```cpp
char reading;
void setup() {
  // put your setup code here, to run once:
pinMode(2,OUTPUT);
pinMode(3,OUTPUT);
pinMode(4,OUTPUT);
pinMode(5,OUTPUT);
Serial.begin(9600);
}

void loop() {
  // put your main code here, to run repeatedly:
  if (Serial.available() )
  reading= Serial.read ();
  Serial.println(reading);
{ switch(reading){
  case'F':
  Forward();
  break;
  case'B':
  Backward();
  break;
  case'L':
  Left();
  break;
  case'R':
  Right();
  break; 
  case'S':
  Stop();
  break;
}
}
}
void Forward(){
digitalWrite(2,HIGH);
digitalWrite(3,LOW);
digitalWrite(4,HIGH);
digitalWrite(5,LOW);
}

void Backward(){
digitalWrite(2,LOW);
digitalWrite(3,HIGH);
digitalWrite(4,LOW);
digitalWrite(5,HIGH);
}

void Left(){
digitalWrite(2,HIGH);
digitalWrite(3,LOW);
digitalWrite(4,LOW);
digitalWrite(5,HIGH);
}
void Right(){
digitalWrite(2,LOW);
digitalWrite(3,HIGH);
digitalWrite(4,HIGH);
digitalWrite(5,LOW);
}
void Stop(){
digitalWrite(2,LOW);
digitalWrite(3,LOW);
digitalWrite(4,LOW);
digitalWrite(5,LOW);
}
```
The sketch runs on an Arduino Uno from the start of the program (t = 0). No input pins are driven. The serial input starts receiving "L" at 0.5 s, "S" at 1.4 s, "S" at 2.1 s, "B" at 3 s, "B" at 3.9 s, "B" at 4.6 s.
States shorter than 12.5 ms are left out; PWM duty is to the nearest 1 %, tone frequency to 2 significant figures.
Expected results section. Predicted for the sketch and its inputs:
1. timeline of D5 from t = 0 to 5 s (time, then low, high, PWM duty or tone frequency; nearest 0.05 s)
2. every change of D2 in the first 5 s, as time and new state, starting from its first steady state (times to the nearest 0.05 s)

0 s low; 0.5 s high; 1.4 s low; 3 s high
0 s low; 0.5 s high; 1.4 s low
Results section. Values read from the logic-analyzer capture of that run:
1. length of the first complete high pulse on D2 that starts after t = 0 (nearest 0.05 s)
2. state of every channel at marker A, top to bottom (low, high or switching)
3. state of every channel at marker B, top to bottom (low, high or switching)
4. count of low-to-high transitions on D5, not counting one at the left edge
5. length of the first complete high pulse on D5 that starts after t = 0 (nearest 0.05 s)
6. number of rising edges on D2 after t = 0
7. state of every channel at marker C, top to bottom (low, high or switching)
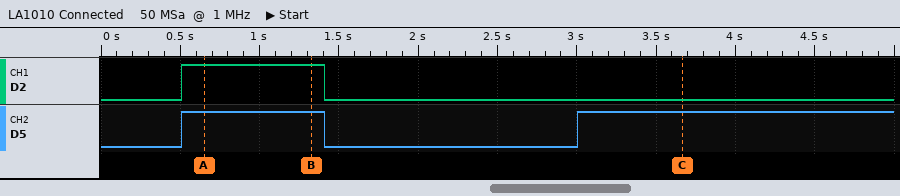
0.90 s
D2 high, D5 high
D2 high, D5 high
2
0.90 s
1
D2 low, D5 high
